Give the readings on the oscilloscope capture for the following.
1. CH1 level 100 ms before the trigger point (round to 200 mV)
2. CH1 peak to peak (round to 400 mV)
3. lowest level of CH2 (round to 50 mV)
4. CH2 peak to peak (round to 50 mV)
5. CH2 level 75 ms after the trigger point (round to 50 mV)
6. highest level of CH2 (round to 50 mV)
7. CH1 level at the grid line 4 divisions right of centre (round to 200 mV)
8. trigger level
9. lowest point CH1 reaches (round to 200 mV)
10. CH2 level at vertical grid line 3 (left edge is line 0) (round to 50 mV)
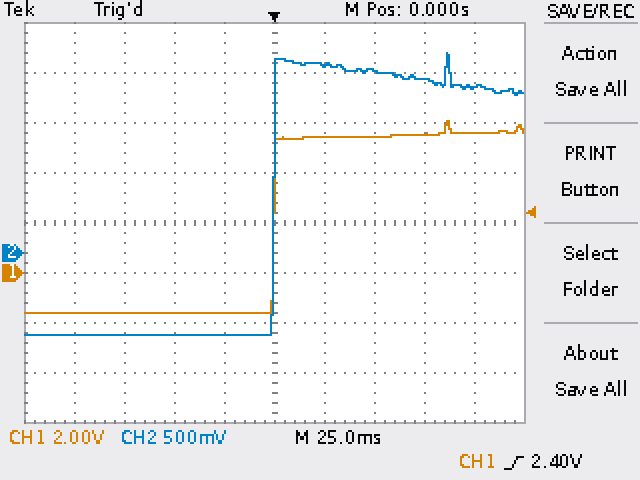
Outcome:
-1.6 V
7.6 V
-800 mV
2.80 V
1.75 V
2.00 V
5.6 V
2.40 V
-1.6 V
-800 mV
